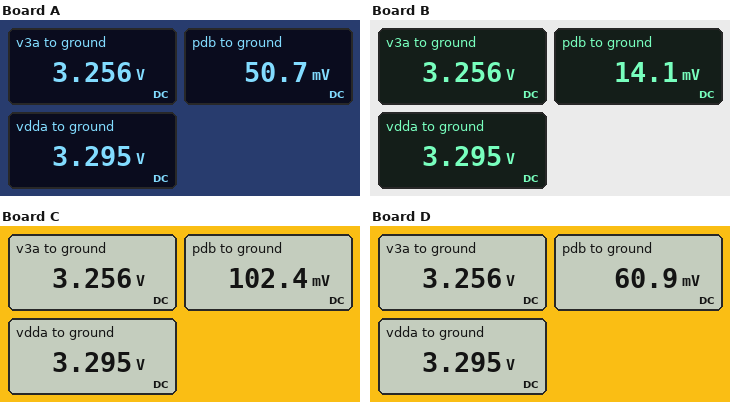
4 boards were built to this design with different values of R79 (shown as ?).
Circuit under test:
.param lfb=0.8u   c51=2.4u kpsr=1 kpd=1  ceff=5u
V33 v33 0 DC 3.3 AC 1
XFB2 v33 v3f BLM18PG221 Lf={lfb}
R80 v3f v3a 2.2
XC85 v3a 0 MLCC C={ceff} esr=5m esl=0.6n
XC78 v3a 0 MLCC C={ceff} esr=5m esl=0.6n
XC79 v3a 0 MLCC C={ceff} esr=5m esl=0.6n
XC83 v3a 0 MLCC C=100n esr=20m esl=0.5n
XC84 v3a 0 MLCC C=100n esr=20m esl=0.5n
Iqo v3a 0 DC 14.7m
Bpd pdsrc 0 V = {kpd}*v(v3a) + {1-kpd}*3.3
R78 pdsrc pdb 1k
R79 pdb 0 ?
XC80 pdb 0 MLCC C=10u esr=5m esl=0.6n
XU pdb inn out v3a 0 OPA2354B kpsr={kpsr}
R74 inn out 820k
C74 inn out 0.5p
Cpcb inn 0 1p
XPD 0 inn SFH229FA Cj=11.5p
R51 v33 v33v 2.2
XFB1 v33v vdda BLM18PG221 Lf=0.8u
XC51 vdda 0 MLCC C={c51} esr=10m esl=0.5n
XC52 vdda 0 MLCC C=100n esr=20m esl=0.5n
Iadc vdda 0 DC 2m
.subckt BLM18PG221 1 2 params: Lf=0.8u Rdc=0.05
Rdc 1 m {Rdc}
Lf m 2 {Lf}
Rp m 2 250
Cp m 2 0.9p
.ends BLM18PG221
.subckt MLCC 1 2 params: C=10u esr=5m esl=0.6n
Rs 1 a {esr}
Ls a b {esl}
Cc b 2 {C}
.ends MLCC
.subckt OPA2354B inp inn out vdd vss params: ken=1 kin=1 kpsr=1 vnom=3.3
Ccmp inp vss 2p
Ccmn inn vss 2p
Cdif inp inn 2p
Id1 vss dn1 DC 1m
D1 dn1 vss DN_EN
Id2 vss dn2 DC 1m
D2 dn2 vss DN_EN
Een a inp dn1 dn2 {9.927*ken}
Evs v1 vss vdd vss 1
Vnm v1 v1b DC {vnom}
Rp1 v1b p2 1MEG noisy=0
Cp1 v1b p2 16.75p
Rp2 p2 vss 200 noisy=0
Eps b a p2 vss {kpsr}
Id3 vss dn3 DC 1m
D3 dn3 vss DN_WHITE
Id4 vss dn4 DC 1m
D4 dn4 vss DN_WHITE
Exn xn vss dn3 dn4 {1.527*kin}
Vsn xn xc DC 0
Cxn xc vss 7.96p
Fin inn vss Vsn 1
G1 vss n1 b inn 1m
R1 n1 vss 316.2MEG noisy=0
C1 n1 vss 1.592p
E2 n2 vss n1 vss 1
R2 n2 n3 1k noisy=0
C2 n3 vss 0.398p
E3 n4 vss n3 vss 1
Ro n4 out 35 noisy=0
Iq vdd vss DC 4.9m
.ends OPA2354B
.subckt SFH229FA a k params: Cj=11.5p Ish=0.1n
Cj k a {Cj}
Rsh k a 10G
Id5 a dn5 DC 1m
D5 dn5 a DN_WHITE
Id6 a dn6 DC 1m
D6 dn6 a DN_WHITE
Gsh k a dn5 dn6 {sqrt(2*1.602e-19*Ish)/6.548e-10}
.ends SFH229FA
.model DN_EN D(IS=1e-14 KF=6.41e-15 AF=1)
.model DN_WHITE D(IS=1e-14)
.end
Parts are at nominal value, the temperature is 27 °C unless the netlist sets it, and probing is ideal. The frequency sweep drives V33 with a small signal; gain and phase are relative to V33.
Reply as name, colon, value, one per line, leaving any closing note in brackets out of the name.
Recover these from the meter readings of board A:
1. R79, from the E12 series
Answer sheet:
R79, from the E12 series: 56 Ω
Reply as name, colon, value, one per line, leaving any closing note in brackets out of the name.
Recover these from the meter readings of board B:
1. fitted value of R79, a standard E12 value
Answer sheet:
fitted value of R79, a standard E12 value: 15 Ω
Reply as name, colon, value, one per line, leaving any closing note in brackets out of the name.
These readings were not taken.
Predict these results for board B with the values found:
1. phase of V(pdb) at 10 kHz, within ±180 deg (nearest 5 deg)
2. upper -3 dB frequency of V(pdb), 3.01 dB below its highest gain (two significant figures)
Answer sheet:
phase of V(pdb) at 10 kHz, within ±180 deg: -150 deg
upper -3 dB frequency of V(pdb), 3.01 dB below its highest gain: 1.0 kHz
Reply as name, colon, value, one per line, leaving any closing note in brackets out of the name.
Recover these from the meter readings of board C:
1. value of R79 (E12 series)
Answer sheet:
value of R79: 120 Ω
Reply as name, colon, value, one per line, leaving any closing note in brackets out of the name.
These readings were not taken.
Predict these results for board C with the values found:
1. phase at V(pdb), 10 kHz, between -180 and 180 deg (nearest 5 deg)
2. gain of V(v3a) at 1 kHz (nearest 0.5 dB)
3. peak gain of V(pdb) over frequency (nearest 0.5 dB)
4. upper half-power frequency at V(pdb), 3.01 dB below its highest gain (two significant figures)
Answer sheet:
phase at V(pdb), 10 kHz, between -180 and 180 deg: -155 deg
gain of V(v3a) at 1 kHz: 0 dB
peak gain of V(pdb) over frequency: -19.5 dB
upper half-power frequency at V(pdb), 3.01 dB below its highest gain: 150 Hz
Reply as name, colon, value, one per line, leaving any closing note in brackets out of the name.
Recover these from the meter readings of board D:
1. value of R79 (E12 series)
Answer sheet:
value of R79: 68 Ω
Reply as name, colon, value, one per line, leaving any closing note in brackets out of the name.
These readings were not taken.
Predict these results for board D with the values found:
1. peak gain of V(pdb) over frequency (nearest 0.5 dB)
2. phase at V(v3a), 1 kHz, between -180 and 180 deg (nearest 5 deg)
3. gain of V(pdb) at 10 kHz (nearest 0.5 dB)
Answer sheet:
peak gain of V(pdb) over frequency: -24.0 dB
phase at V(v3a), 1 kHz, between -180 and 180 deg: -10 deg
gain of V(pdb) at 10 kHz: -63.5 dB
